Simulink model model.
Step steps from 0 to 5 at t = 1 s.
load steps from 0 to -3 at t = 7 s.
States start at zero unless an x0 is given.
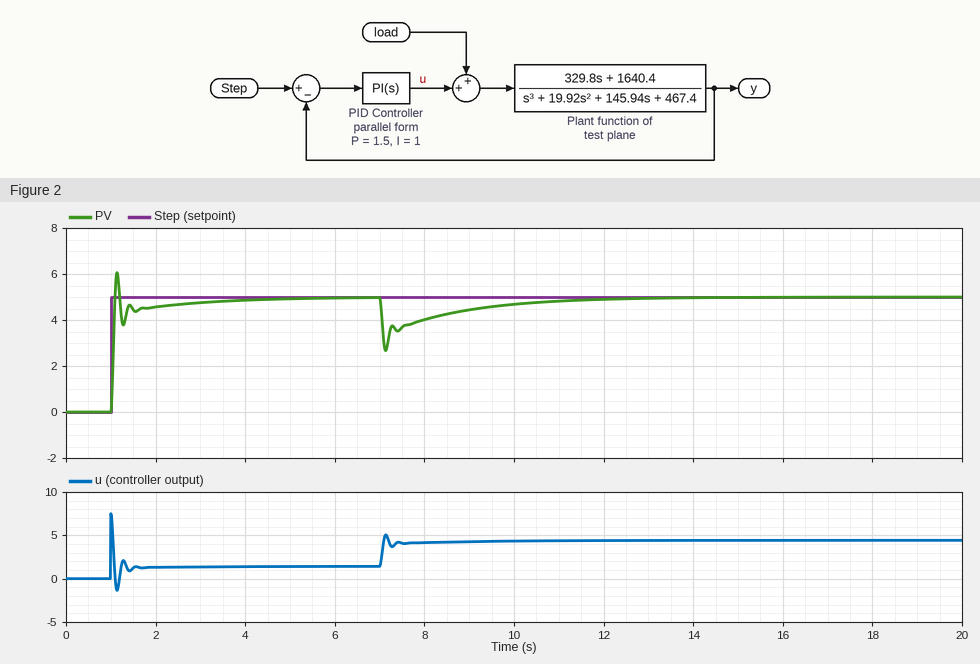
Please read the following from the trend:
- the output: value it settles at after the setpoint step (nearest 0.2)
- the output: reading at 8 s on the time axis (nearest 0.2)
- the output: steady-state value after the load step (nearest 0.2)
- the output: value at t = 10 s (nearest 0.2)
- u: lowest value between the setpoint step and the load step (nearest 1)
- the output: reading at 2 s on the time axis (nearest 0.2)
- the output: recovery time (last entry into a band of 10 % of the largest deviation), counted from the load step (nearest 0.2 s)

5.0
4.0
5.0
4.6
-1
4.6
3.6 s
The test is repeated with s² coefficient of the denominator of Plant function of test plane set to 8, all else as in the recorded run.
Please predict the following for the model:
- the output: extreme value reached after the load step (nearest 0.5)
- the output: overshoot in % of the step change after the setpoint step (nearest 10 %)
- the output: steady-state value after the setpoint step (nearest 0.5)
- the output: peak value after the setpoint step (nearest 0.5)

2.0
50 %
5.0
7.5
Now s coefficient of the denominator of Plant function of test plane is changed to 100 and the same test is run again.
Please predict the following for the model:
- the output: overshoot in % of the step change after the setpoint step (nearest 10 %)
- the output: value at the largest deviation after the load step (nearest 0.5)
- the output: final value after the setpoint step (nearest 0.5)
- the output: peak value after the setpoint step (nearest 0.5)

30 %
2.5
5.0
6.5
